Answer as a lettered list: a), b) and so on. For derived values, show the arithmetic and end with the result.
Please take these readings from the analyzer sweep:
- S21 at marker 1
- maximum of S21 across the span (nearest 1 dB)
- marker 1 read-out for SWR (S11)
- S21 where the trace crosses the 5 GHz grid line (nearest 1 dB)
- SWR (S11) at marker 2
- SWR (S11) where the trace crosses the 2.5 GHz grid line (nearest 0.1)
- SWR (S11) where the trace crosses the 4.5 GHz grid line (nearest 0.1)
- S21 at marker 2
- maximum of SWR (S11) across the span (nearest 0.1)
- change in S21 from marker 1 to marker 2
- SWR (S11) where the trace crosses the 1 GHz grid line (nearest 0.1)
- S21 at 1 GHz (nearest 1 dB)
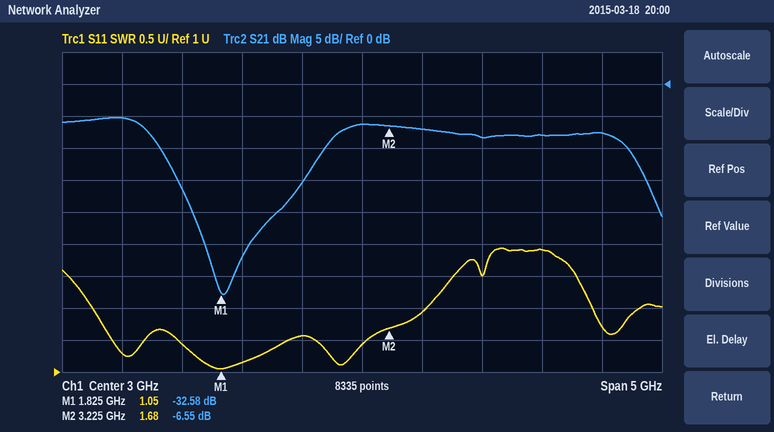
a) -32.58 dB
b) -5 dB
c) 1.05
d) -8 dB
e) 1.68
f) 1.6
g) 2.9
h) -6.55 dB
i) 2.9
j) -6.55 − (-32.58) = 26.03 dB
k) 1.3
l) -5 dB
